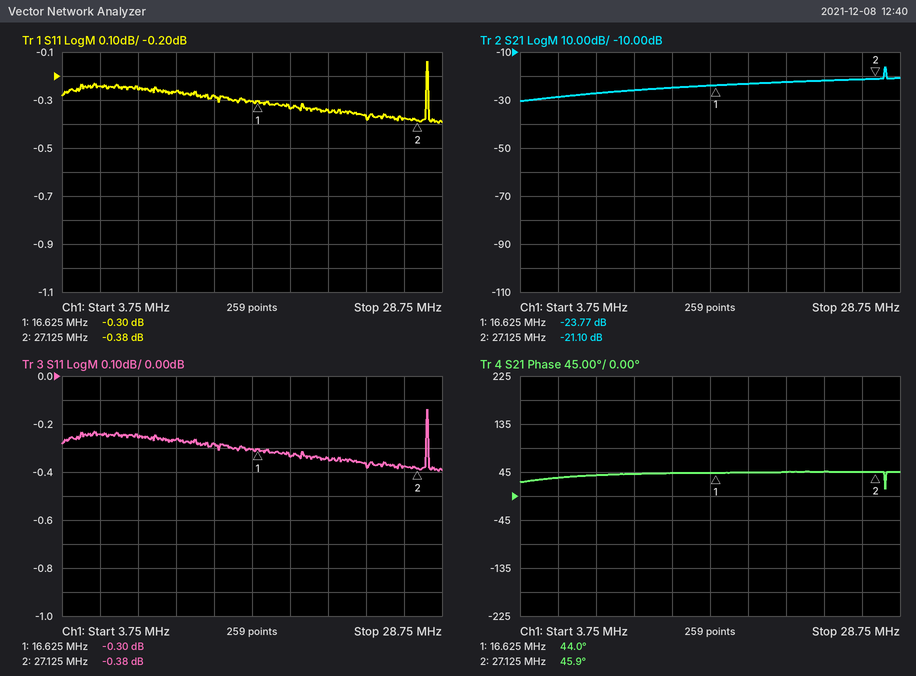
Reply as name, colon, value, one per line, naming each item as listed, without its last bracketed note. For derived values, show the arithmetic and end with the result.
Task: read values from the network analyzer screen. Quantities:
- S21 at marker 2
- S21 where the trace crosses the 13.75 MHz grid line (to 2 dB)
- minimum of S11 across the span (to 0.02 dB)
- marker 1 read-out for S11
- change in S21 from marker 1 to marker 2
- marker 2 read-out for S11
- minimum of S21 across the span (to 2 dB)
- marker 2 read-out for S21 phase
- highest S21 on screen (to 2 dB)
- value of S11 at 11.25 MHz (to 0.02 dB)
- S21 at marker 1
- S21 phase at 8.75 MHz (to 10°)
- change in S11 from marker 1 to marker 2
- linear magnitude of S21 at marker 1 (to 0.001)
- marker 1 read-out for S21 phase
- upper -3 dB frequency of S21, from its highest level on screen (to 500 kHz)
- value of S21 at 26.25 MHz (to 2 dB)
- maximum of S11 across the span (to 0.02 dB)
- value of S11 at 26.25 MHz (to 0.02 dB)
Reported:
S21 at marker 2: -21.10 dB
S21 where the trace crosses the 13.75 MHz grid line: -24 dB
minimum of S11 across the span: -0.40 dB
marker 1 read-out for S11: -0.30 dB
change in S21 from marker 1 to marker 2: -21.1 − (-23.77) = 2.67 dB
marker 2 read-out for S11: -0.38 dB
minimum of S21 across the span: -30 dB
marker 2 read-out for S21 phase: 45.9°
highest S21 on screen: -16 dB
value of S11 at 11.25 MHz: -0.26 dB
S21 at marker 1: -23.77 dB
S21 phase at 8.75 MHz: 40°
change in S11 from marker 1 to marker 2: -0.38 − (-0.3) = -0.08 dB
linear magnitude of S21 at marker 1: 10^(-23.77/20) ≈ 0.065
marker 1 read-out for S21 phase: 44.0°
upper -3 dB frequency of S21, from its highest level on screen: 28.0 MHz
value of S21 at 26.25 MHz: -22 dB
maximum of S11 across the span: -0.14 dB
value of S11 at 26.25 MHz: -0.38 dB
